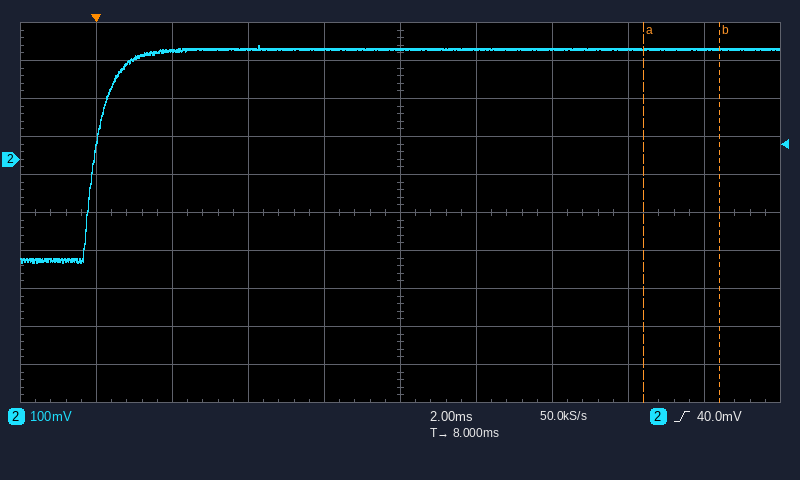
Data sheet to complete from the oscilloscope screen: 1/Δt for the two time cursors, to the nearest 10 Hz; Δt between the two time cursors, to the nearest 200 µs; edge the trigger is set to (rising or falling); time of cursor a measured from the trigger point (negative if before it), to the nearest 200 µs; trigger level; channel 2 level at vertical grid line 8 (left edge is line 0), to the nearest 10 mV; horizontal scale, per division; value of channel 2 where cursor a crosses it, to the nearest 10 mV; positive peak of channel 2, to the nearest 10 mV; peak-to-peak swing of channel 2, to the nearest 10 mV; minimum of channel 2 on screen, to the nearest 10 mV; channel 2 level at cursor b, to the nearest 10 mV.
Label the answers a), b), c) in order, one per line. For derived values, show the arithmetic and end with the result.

a) 1 / 2.0 ms ≈ 500 Hz
b) 2.0 ms
c) rising
d) +14.4 ms
e) 40.0 mV
f) 290 mV
g) 2 ms
h) 290 mV
i) 300 mV
j) 300 mV − (-270 mV) = 570 mV
k) -270 mV
l) 290 mV
